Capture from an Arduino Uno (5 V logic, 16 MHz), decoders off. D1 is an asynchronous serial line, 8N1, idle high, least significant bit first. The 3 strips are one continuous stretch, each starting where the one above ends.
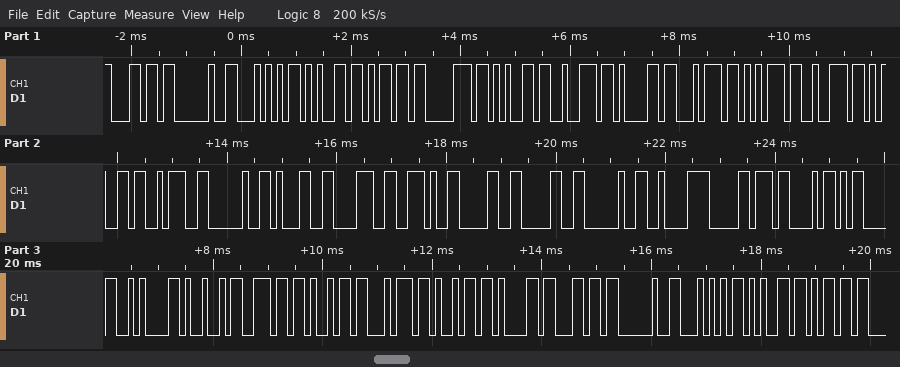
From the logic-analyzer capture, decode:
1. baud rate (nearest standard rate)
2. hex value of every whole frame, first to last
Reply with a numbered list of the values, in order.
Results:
1. 9600 baud
2. 6C 20 54 65 6D 70 65 72 61 74 75 72 65 3A 20 31 38 2E 30 30 20 C2 B0 43 0D 0A 49 6E 69 74 69 61 6C 20 54 65 6D
